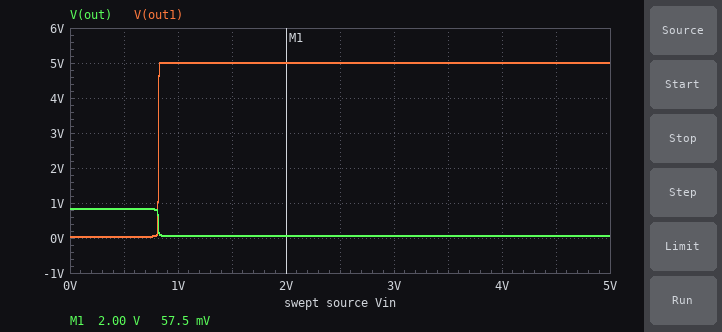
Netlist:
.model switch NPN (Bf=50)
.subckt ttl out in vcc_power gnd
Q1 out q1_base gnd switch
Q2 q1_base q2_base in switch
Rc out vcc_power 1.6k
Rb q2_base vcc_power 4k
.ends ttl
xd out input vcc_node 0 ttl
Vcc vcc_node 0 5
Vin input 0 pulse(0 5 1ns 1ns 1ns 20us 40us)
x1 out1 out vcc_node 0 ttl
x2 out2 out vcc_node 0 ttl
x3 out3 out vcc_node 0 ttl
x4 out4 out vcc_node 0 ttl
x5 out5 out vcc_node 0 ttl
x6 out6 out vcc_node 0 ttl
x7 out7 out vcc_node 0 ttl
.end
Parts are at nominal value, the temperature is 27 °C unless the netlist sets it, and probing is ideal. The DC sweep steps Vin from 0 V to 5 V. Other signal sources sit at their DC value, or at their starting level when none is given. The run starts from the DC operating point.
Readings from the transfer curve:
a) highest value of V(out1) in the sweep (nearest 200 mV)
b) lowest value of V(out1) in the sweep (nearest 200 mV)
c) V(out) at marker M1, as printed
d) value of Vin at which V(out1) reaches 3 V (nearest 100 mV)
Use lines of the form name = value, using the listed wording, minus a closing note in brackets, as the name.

highest value of V(out1) in the sweep = 5.0 V
lowest value of V(out1) in the sweep = 0 V
V(out) at marker M1, as printed = 57.5 mV
value of Vin at which V(out1) reaches 3 V = 800 mV
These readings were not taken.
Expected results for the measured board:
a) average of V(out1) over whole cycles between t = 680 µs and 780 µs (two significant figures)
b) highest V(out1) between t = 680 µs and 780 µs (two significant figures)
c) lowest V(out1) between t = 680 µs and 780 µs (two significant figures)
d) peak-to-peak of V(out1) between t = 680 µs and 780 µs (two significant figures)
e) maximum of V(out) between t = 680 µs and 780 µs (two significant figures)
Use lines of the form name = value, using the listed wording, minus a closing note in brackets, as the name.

average of V(out1) over whole cycles between t = 680 µs and 780 µs = 2.5 V
highest V(out1) between t = 680 µs and 780 µs = 5.0 V
lowest V(out1) between t = 680 µs and 780 µs = 40 mV
peak-to-peak of V(out1) between t = 680 µs and 780 µs = 5.0 V
maximum of V(out) between t = 680 µs and 780 µs = 830 mV
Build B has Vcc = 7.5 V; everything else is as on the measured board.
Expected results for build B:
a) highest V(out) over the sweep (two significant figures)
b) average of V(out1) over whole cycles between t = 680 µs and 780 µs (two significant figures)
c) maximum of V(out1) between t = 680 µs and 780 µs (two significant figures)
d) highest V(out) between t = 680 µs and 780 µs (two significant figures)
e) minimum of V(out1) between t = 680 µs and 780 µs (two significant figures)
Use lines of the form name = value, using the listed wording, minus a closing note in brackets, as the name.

highest V(out) over the sweep = 840 mV
average of V(out1) over whole cycles between t = 680 µs and 780 µs = 3.8 V
maximum of V(out1) between t = 680 µs and 780 µs = 7.5 V
highest V(out) between t = 680 µs and 780 µs = 840 mV
minimum of V(out1) between t = 680 µs and 780 µs = 39 mV
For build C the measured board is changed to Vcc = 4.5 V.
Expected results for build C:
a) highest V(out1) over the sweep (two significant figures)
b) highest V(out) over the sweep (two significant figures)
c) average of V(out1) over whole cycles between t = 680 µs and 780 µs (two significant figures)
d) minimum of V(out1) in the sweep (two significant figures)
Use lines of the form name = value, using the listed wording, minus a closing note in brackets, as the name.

highest V(out1) over the sweep = 4.5 V
highest V(out) over the sweep = 830 mV
average of V(out1) over whole cycles between t = 680 µs and 780 µs = 2.3 V
minimum of V(out1) in the sweep = 41 mV
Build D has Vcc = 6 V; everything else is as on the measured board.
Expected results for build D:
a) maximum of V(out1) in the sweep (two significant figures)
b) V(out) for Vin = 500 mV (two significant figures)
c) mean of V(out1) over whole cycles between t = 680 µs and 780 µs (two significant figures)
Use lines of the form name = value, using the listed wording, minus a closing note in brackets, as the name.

maximum of V(out1) in the sweep = 6.0 V
V(out) for Vin = 500 mV = 840 mV
mean of V(out1) over whole cycles between t = 680 µs and 780 µs = 3.0 V
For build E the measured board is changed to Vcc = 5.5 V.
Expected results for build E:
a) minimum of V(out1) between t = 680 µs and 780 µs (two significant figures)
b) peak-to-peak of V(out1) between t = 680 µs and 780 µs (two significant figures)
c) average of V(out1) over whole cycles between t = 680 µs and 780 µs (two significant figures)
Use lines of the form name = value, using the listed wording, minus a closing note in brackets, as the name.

minimum of V(out1) between t = 680 µs and 780 µs = 40 mV
peak-to-peak of V(out1) between t = 680 µs and 780 µs = 5.5 V
average of V(out1) over whole cycles between t = 680 µs and 780 µs = 2.8 V
